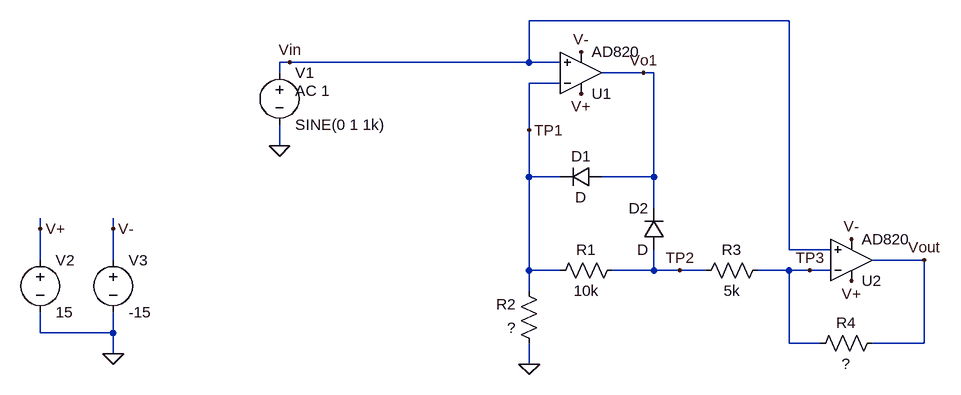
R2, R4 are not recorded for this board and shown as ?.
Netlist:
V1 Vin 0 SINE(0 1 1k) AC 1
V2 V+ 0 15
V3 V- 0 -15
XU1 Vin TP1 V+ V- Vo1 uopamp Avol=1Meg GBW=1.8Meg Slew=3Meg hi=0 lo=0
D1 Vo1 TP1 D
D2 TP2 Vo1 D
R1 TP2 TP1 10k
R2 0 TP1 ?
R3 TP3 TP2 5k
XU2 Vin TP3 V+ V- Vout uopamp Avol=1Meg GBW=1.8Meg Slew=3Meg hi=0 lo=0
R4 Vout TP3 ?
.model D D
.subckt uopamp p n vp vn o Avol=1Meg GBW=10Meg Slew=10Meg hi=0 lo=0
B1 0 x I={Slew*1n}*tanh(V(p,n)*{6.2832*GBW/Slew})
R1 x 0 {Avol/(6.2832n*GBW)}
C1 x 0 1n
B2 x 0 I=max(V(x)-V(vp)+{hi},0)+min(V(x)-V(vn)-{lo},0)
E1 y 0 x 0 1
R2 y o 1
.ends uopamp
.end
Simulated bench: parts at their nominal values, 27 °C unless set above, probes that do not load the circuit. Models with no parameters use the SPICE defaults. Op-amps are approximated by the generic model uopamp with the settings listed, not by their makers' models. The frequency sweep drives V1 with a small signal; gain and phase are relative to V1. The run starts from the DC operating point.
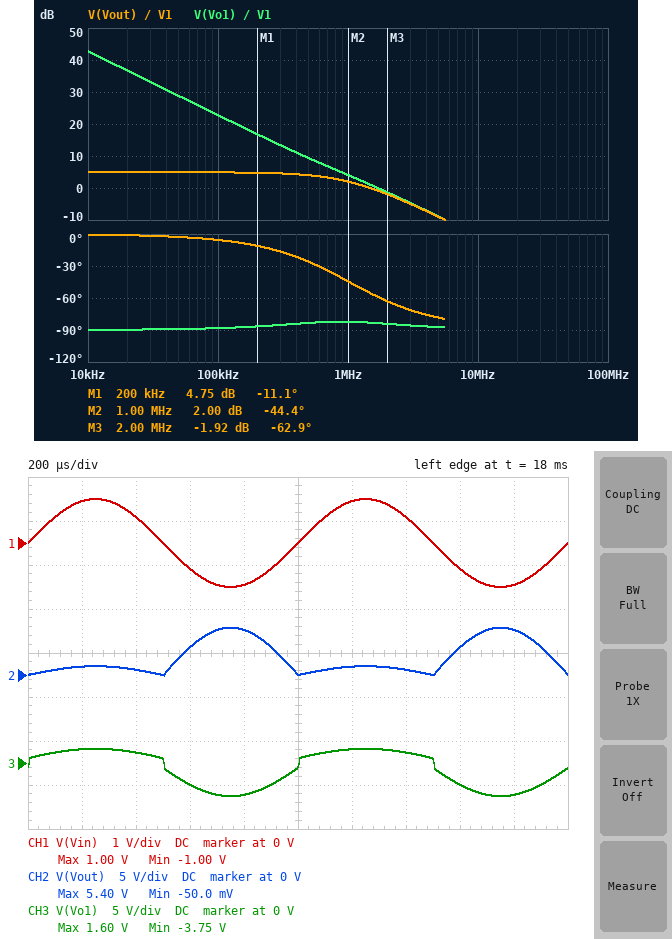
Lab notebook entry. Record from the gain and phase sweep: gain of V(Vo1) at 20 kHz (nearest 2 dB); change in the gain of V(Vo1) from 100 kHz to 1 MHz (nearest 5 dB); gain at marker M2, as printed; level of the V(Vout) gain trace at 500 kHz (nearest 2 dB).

36 dB
-20 dB
2.00 dB
4 dB
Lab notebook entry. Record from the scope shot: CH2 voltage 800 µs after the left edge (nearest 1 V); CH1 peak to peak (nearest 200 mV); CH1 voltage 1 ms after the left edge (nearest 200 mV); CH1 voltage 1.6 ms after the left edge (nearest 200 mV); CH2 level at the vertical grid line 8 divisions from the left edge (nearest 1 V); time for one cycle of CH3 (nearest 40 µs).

5 V
2.0 V
0 V
-600 mV
3 V
1.00 ms
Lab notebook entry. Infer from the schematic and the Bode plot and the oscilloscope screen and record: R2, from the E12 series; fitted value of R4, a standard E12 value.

4.7 kΩ
15 kΩ
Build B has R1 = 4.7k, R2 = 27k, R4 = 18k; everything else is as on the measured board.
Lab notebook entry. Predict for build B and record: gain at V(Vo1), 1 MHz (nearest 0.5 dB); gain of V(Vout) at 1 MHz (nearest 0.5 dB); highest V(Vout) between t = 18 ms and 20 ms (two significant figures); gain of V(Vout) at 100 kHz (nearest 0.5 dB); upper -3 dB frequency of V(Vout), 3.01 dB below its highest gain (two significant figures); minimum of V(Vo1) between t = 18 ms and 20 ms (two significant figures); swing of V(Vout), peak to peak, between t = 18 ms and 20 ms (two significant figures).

1.5 dB
1.0 dB
1.0 V
3.5 dB
1.2 MHz
-1.8 V
1.4 V
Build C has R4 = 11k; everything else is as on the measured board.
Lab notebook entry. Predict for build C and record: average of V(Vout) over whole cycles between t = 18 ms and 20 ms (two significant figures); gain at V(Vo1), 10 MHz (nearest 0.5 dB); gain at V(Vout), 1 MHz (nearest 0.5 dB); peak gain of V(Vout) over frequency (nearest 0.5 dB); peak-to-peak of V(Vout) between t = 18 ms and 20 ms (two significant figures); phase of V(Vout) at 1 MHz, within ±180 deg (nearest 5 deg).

1.5 V
-15.0 dB
1.5 dB
4.0 dB
3.7 V
-40 deg
